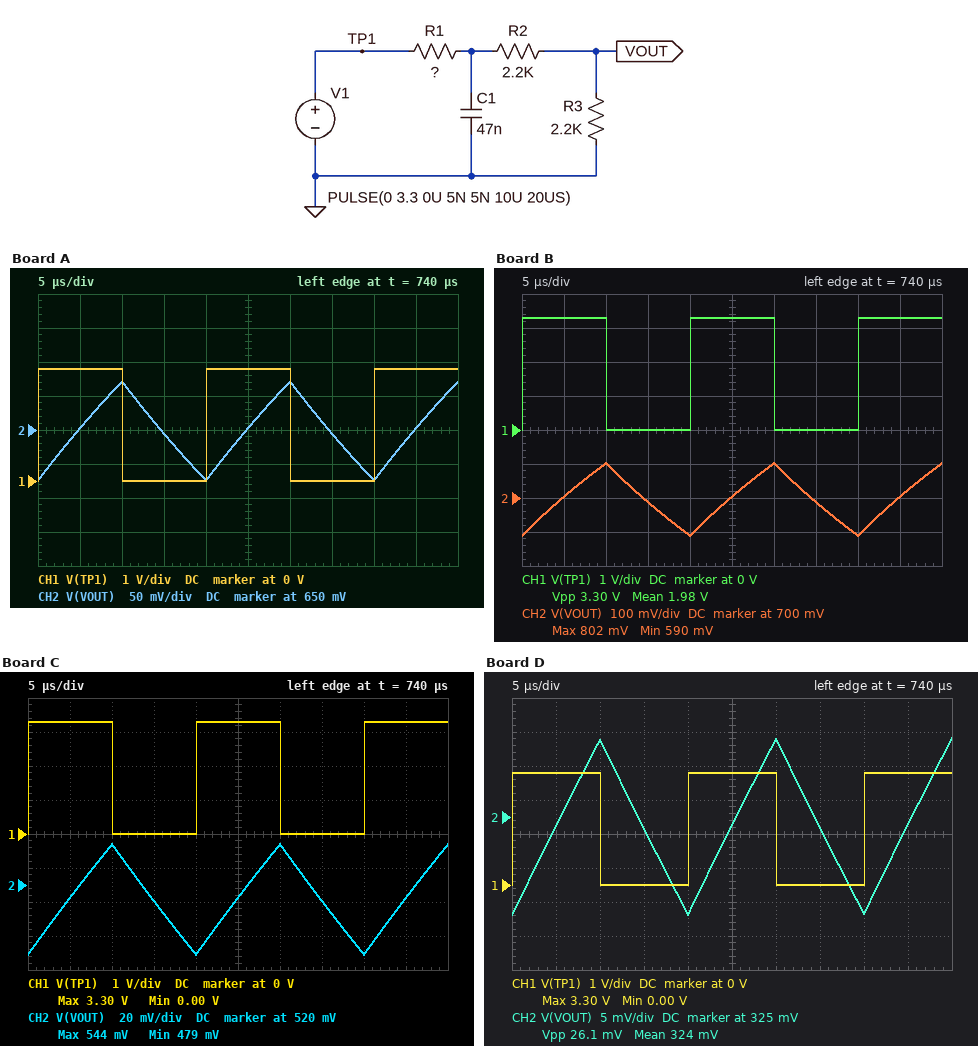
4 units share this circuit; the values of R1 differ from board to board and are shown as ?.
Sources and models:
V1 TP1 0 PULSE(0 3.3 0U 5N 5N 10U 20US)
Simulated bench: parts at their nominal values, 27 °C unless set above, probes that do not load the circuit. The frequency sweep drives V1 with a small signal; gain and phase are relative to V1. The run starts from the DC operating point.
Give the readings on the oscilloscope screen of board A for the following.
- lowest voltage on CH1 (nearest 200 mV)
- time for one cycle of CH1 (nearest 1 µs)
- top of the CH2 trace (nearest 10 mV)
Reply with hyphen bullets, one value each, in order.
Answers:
- 0 V
- 20 µs
- 720 mV
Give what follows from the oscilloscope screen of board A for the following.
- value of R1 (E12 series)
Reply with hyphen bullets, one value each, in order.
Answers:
- 1.2 kΩ
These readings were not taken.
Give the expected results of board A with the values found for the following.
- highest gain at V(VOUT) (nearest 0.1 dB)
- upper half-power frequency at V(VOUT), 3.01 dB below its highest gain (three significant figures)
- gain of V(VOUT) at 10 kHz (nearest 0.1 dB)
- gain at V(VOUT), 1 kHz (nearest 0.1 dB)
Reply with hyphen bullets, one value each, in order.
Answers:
- -8.1 dB
- 3.59 kHz
- -17.5 dB
- -8.4 dB
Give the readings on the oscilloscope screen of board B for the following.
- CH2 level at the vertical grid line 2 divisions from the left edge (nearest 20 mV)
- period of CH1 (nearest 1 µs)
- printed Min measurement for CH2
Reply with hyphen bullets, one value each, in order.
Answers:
- 800 mV
- 20 µs
- 590 mV
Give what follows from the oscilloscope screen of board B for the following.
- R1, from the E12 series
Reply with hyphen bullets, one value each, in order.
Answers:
- 820 Ω
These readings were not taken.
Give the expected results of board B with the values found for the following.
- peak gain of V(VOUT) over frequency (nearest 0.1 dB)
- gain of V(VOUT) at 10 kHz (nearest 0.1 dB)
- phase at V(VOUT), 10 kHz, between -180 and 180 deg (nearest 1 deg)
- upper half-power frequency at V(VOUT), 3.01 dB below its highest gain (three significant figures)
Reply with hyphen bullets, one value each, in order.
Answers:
- -7.5 dB
- -14.6 dB
- -64 deg
- 4.90 kHz
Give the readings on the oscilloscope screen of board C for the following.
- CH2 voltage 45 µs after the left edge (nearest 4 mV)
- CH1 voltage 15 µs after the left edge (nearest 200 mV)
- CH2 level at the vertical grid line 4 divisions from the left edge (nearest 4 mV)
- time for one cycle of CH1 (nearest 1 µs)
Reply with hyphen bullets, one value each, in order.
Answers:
- 512 mV
- 0 V
- 480 mV
- 20 µs
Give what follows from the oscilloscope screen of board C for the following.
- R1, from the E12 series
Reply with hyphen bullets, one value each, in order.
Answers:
- 2.7 kΩ
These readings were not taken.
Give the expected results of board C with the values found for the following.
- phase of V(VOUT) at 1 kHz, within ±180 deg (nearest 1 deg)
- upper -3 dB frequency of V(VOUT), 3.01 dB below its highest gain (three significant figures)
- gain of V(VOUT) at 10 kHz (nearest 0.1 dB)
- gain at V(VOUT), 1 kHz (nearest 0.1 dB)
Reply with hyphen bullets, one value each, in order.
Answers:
- -26 deg
- 2.02 kHz
- -24.2 dB
- -11.1 dB
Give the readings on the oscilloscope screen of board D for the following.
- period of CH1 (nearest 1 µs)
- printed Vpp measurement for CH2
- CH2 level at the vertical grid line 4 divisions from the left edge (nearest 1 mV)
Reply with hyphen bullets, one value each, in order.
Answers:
- 20 µs
- 26.1 mV
- 311 mV
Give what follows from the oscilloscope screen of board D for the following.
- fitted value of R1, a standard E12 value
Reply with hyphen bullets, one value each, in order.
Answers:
- 6.8 kΩ
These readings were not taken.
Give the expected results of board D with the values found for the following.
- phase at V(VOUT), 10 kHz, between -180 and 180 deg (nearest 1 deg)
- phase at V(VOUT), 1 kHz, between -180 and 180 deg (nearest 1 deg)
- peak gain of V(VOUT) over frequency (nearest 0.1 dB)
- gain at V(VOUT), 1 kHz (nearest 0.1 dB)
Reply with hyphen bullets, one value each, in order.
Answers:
- -83 deg
- -38 deg
- -14.1 dB
- -16.2 dB
